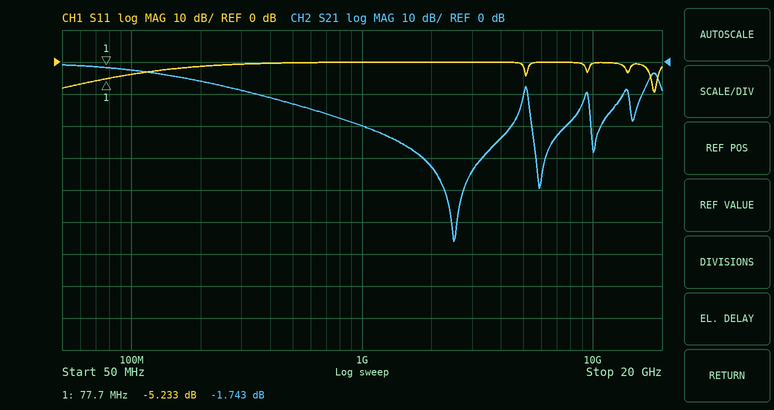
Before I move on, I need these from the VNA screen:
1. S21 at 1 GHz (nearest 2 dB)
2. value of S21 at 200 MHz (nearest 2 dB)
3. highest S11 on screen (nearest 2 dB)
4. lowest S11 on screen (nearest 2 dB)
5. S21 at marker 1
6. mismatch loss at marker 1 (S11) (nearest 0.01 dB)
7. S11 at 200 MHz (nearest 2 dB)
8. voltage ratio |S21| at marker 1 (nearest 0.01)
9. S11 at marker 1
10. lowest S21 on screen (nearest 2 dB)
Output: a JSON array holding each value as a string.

["-20 dB", "-6 dB", "0 dB", "-10 dB", "-1.743 dB", "1.55 dB", "-2 dB", "0.82", "-5.233 dB", "-56 dB"]
